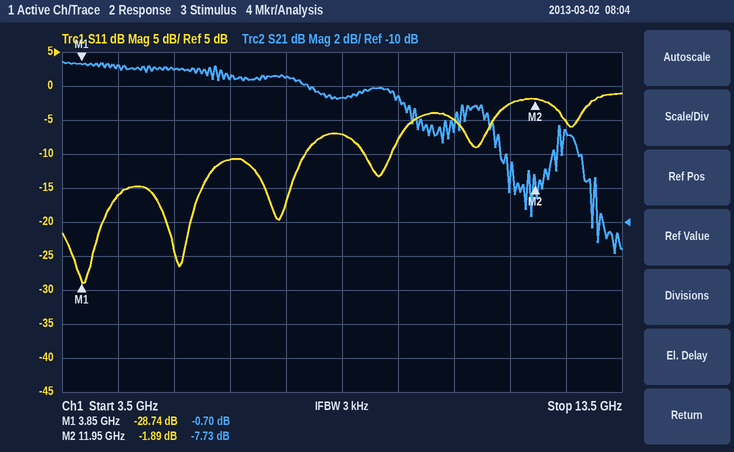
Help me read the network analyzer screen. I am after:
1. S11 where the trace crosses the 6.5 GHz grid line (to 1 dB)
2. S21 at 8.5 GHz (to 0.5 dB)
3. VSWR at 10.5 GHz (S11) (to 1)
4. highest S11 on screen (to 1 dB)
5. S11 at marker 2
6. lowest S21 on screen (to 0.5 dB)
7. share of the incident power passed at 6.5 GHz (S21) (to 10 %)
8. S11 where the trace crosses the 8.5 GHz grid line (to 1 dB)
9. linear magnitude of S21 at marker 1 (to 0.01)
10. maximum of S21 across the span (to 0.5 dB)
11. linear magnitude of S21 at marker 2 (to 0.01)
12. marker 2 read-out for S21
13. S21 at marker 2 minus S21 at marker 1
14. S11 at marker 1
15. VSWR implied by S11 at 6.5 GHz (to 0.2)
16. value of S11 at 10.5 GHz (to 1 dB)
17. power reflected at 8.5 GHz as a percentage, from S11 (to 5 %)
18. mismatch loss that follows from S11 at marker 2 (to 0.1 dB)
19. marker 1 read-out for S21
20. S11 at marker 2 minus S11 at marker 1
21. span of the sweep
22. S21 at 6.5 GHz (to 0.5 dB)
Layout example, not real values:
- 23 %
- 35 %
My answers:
- -11 dB
- -2.5 dB
- 4
- -1 dB
- -1.89 dB
- -12.0 dB
- 70 %
- -7 dB
- 0.92
- -0.5 dB
- 0.41
- -7.73 dB
- -7.03 dB
- -28.74 dB
- 1.8
- -5 dB
- 20 %
- 4.5 dB
- -0.70 dB
- 26.85 dB
- 10 GHz
- -1.5 dB
